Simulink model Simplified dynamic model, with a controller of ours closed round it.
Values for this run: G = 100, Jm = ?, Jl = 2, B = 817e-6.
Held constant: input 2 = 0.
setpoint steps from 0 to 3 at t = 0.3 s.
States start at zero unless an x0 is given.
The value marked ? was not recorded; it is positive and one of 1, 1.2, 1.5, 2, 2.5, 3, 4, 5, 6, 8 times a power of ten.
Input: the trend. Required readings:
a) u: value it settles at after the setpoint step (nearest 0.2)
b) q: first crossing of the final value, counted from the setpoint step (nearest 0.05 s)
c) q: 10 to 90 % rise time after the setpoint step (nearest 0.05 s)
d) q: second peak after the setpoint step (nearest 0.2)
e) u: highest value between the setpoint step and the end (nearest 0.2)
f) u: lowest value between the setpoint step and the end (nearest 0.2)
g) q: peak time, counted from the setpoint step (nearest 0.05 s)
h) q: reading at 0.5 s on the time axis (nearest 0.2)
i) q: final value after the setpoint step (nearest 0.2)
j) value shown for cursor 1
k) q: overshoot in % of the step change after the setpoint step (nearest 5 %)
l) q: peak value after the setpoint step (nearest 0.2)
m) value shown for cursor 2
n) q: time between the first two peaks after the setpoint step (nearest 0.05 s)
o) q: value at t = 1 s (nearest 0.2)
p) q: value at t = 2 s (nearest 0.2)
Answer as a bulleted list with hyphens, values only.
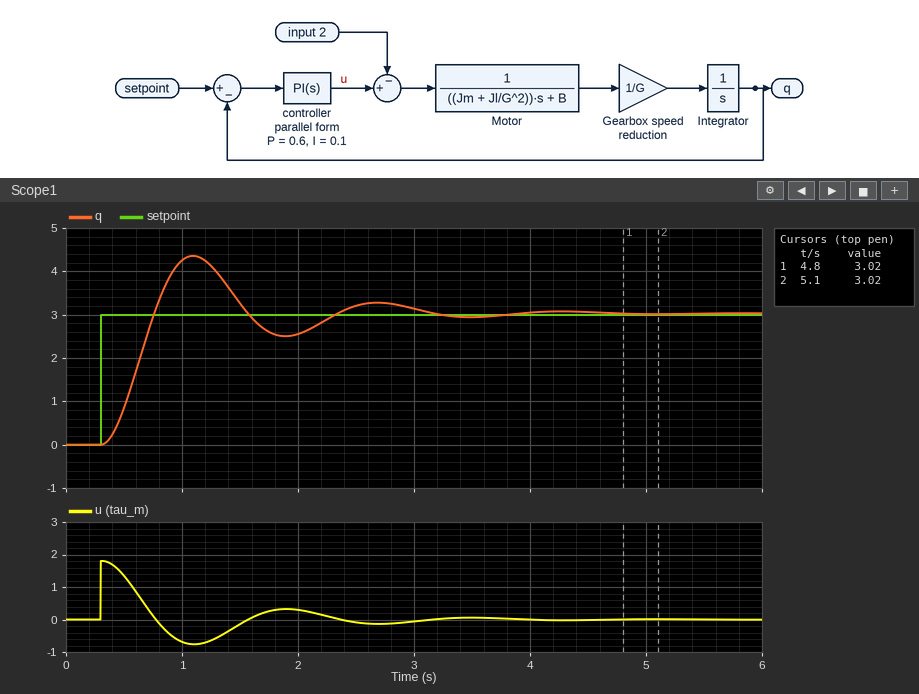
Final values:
- 0.0
- 0.45 s
- 0.30 s
- 3.2
- 1.8
- -0.8
- 0.80 s
- 0.8
- 3.0
- 3.02
- 45 %
- 4.4
- 3.02
- 1.60 s
- 4.2
- 2.6
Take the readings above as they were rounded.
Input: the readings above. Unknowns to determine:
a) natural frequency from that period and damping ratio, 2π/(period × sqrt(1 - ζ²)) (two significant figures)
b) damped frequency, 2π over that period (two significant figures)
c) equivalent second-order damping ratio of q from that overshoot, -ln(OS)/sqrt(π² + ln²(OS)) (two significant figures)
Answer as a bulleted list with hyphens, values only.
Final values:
- 4.1 rad/s
- 3.9 rad/s
- 0.25
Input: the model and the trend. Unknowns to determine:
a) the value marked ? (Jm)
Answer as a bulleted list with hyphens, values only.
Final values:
- 0.00015
